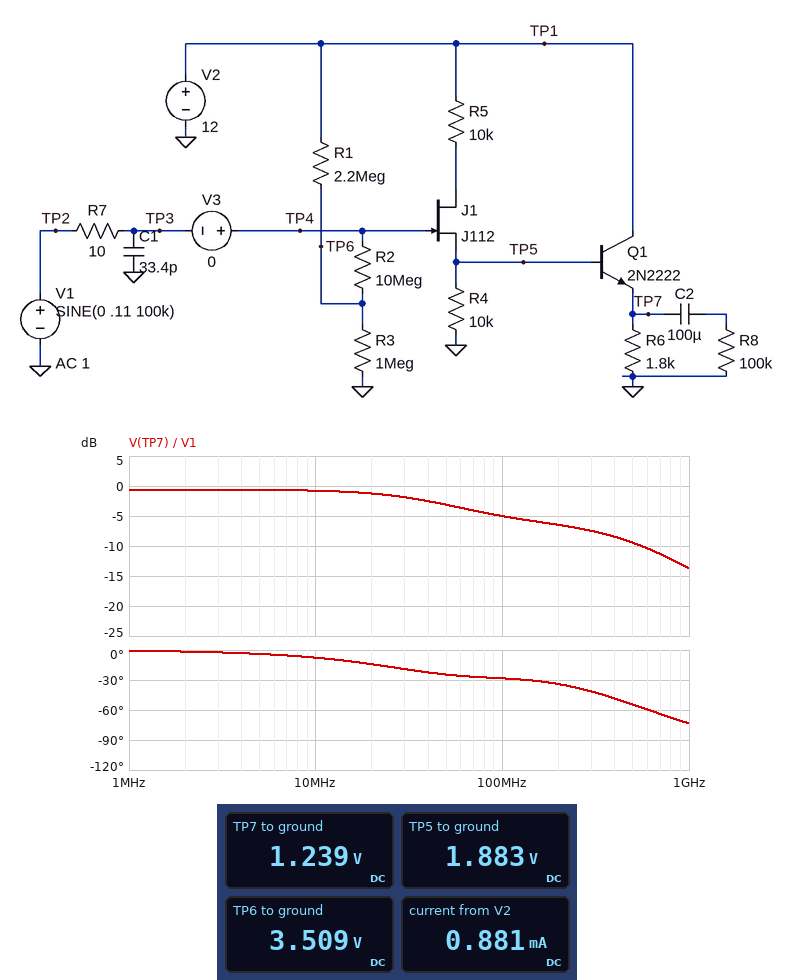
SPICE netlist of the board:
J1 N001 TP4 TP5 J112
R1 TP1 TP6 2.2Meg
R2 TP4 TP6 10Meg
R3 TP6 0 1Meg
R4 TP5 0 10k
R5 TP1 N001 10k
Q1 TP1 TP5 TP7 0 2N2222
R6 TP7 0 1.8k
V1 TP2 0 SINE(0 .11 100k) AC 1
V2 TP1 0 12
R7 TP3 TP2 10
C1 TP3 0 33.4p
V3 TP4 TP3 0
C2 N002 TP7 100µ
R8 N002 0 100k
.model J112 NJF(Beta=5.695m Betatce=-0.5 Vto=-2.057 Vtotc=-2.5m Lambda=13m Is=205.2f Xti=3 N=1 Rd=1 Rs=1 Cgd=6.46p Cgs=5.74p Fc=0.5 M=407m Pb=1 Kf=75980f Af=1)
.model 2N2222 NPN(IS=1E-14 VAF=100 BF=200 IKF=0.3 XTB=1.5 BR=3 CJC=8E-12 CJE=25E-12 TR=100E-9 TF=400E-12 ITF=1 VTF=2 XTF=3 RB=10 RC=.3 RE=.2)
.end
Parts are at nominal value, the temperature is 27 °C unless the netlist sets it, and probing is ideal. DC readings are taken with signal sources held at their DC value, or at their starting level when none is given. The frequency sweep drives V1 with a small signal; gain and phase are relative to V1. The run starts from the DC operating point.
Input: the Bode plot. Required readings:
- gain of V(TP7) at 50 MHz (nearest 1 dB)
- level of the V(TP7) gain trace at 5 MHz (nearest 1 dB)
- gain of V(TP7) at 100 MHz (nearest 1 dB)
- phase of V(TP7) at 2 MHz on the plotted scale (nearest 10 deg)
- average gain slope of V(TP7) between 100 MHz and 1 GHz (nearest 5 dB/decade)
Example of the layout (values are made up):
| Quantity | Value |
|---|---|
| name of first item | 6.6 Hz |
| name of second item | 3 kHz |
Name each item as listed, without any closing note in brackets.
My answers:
| Quantity | Value |
|---|---|
| gain of V(TP7) at 50 MHz | -3 dB |
| level of the V(TP7) gain trace at 5 MHz | -1 dB |
| gain of V(TP7) at 100 MHz | -5 dB |
| phase of V(TP7) at 2 MHz on the plotted scale | 0 deg |
| average gain slope of V(TP7) between 100 MHz and 1 GHz | -10 dB/decade |
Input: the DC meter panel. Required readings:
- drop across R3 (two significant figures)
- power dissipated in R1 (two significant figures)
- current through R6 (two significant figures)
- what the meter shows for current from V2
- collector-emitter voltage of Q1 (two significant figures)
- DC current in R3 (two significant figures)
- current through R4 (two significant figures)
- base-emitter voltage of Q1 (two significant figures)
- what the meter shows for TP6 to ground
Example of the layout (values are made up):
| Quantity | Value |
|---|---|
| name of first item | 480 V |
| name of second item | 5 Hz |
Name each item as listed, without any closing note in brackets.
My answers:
| Quantity | Value |
|---|---|
| drop across R3 | 3.5 V |
| power dissipated in R1 | 33 µW |
| current through R6 | 690 µA |
| what the meter shows for current from V2 | 0.881 mA |
| collector-emitter voltage of Q1 | 11 V |
| DC current in R3 | 3.5 µA |
| current through R4 | 190 µA |
| base-emitter voltage of Q1 | 640 mV |
| what the meter shows for TP6 to ground | 3.509 V |
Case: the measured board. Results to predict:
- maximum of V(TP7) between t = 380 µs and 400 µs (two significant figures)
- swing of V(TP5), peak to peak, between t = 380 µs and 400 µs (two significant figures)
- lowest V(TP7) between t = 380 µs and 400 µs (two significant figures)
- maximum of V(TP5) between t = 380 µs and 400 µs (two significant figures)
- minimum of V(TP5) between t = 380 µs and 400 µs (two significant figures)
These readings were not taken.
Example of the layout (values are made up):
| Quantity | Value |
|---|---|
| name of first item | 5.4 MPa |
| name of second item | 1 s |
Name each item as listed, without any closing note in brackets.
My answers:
| Quantity | Value |
|---|---|
| maximum of V(TP7) between t = 380 µs and 400 µs | 1.3 V |
| swing of V(TP5), peak to peak, between t = 380 µs and 400 µs | 210 mV |
| lowest V(TP7) between t = 380 µs and 400 µs | 1.1 V |
| maximum of V(TP5) between t = 380 µs and 400 µs | 2.0 V |
| minimum of V(TP5) between t = 380 µs and 400 µs | 1.8 V |
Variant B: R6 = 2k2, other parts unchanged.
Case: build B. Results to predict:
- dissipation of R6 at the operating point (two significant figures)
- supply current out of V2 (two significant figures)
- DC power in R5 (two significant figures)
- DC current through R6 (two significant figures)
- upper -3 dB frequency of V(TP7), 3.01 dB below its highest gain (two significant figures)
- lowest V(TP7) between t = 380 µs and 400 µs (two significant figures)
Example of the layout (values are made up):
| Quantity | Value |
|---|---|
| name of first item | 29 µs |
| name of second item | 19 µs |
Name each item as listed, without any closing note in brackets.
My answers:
| Quantity | Value |
|---|---|
| dissipation of R6 at the operating point | 700 µW |
| supply current out of V2 | 760 µA |
| DC power in R5 | 360 µW |
| DC current through R6 | 570 µA |
| upper -3 dB frequency of V(TP7), 3.01 dB below its highest gain | 61 MHz |
| lowest V(TP7) between t = 380 µs and 400 µs | 1.1 V |
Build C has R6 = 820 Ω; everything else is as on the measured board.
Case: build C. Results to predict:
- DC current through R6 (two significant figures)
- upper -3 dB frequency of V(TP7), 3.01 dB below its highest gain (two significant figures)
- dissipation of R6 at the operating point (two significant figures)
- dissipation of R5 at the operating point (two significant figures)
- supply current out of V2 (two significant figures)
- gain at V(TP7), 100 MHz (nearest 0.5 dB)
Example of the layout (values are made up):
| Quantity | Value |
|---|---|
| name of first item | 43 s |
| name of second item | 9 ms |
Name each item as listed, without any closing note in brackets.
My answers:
| Quantity | Value |
|---|---|
| DC current through R6 | 1.5 mA |
| upper -3 dB frequency of V(TP7), 3.01 dB below its highest gain | 55 MHz |
| dissipation of R6 at the operating point | 1.8 mW |
| dissipation of R5 at the operating point | 380 µW |
| supply current out of V2 | 1.7 mA |
| gain at V(TP7), 100 MHz | -5.5 dB |
